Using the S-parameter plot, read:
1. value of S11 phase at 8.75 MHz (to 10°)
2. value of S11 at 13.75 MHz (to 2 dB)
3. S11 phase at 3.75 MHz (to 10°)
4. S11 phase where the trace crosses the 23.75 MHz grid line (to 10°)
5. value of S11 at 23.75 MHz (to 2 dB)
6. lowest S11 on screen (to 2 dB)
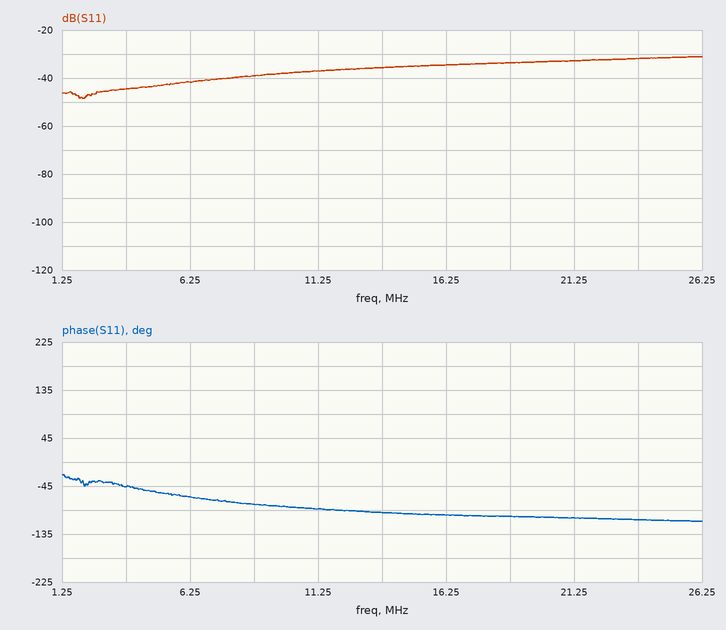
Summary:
-80°
-36 dB
-50°
-110°
-32 dB
-48 dB
